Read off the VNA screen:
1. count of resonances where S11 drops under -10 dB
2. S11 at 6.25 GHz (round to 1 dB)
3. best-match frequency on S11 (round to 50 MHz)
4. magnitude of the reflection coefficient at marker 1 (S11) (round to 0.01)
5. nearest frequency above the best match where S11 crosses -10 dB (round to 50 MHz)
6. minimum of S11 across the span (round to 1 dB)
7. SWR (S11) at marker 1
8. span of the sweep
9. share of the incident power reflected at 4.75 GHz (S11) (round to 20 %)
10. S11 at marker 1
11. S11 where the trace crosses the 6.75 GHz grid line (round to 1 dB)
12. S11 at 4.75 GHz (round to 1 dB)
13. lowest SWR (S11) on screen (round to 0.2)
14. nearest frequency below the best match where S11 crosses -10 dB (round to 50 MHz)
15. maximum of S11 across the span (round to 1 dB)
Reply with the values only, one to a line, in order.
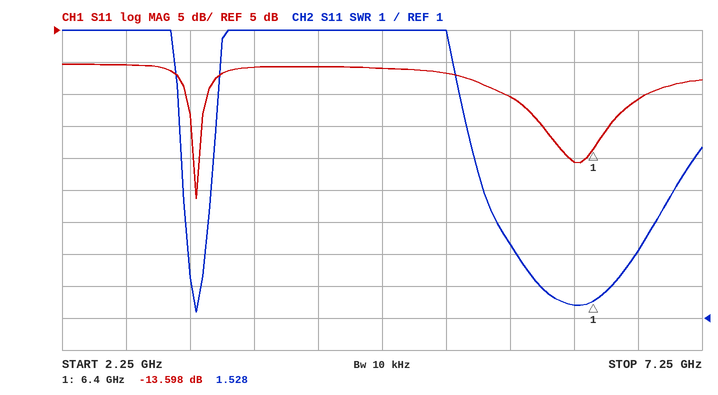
2
-16 dB
3.30 GHz
0.21
3.35 GHz
-21 dB
1.528
5 GHz
80 %
-13.598 dB
-6 dB
-1 dB
1.2
3.25 GHz
0 dB
